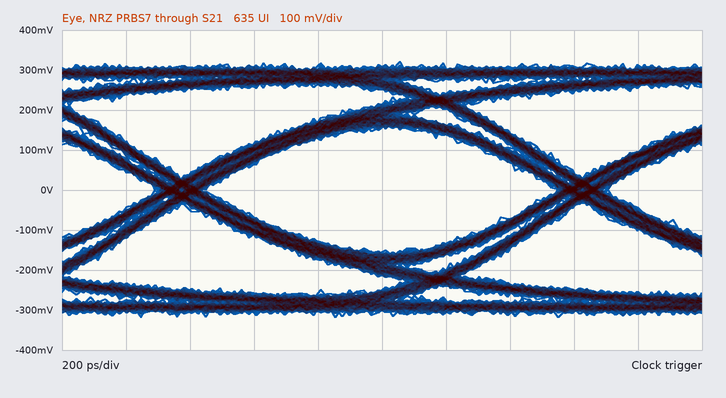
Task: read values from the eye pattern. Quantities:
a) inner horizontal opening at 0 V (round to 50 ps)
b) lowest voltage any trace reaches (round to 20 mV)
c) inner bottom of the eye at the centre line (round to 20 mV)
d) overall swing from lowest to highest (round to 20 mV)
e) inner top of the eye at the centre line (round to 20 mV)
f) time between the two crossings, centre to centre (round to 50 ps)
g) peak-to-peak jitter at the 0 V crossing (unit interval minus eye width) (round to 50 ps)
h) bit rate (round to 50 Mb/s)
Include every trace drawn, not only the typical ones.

1.10 ns
-320 mV
-160 mV
640 mV
160 mV
1.25 ns
150 ps
800 Mb/s
